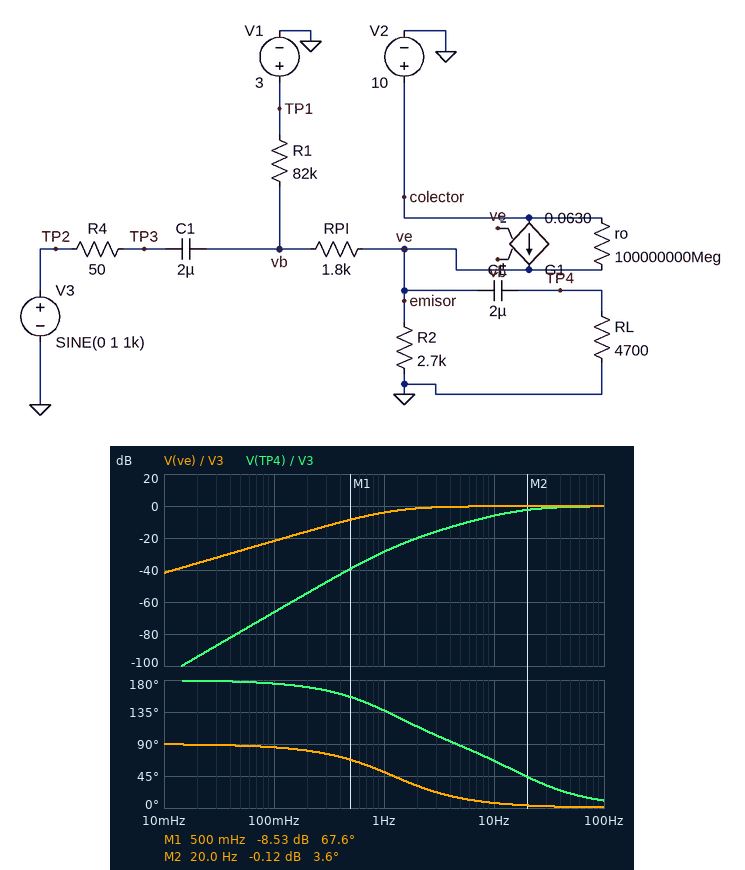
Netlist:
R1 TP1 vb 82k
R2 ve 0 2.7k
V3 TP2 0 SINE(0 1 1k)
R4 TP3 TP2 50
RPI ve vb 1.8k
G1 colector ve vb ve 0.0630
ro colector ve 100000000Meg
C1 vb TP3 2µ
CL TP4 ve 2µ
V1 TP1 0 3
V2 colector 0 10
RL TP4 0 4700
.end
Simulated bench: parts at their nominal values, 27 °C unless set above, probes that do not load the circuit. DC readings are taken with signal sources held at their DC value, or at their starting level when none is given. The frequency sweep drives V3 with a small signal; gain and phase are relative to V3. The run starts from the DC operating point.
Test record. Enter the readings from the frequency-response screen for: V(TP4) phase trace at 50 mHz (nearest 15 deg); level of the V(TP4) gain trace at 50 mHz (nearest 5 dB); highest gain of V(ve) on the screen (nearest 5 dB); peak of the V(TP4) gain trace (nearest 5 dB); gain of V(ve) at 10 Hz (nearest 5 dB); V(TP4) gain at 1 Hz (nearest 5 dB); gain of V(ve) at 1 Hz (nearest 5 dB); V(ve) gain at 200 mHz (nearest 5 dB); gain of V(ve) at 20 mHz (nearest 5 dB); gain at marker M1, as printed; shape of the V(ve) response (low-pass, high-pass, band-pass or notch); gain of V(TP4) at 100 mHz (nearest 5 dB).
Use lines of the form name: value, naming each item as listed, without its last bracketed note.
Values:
V(TP4) phase trace at 50 mHz: 180 deg
level of the V(TP4) gain trace at 50 mHz: -80 dB
highest gain of V(ve) on the screen: 0 dB
peak of the V(TP4) gain trace: 0 dB
gain of V(ve) at 10 Hz: 0 dB
V(TP4) gain at 1 Hz: -30 dB
gain of V(ve) at 1 Hz: -5 dB
V(ve) gain at 200 mHz: -15 dB
gain of V(ve) at 20 mHz: -35 dB
gain at marker M1, as printed: -8.53 dB
shape of the V(ve) response: high-pass
gain of V(TP4) at 100 mHz: -65 dB
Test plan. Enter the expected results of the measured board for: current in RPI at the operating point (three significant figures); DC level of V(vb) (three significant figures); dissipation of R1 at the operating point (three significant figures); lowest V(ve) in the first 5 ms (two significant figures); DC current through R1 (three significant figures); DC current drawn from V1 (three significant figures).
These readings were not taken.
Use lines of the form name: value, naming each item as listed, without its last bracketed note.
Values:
current in RPI at the operating point: 7.64 µA
DC level of V(vb): 2.37 V
dissipation of R1 at the operating point: 4.79 µW
lowest V(ve) in the first 5 ms: 1.4 V
DC current through R1: 7.64 µA
DC current drawn from V1: 7.64 µA
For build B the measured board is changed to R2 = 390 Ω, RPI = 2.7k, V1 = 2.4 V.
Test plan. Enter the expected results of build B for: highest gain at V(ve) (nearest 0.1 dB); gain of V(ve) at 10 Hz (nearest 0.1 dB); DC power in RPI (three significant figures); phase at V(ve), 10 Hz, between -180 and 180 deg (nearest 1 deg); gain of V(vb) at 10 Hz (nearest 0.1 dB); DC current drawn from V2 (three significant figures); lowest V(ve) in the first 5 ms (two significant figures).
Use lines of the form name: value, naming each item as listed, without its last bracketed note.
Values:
highest gain at V(ve): -0.4 dB
gain of V(ve) at 10 Hz: -0.6 dB
DC power in RPI: 678 nW
phase at V(ve), 10 Hz, between -180 and 180 deg: 12 deg
gain of V(vb) at 10 Hz: -0.2 dB
DC current drawn from V2: 2.70 mA
lowest V(ve) in the first 5 ms: 99 mV
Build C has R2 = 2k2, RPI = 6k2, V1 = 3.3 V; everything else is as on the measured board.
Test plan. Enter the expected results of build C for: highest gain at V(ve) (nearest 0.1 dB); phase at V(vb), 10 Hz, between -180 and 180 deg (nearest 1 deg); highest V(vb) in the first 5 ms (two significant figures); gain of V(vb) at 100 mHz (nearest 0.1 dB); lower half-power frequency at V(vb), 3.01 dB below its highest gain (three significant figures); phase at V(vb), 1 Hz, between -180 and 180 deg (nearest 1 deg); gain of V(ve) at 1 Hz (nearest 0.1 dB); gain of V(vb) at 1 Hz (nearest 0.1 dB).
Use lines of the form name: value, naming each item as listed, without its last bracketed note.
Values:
highest gain at V(ve): -0.1 dB
phase at V(vb), 10 Hz, between -180 and 180 deg: 6 deg
highest V(vb) in the first 5 ms: 4.0 V
gain of V(vb) at 100 mHz: -20.6 dB
lower half-power frequency at V(vb), 3.01 dB below its highest gain: 1.06 Hz
phase at V(vb), 1 Hz, between -180 and 180 deg: 47 deg
gain of V(ve) at 1 Hz: -3.4 dB
gain of V(vb) at 1 Hz: -3.3 dB
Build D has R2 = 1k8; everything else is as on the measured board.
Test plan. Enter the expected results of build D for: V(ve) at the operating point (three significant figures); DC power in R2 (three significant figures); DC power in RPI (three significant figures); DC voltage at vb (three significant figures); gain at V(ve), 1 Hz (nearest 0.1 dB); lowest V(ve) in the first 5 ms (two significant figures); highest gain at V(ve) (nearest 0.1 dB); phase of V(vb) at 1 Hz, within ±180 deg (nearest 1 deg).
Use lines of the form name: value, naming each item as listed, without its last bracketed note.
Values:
V(ve) at the operating point: 2.13 V
DC power in R2: 2.53 mW
DC power in RPI: 193 nW
DC voltage at vb: 2.15 V
gain at V(ve), 1 Hz: -4.6 dB
lowest V(ve) in the first 5 ms: 1.1 V
highest gain at V(ve): -0.1 dB
phase of V(vb) at 1 Hz, within ±180 deg: 53 deg
